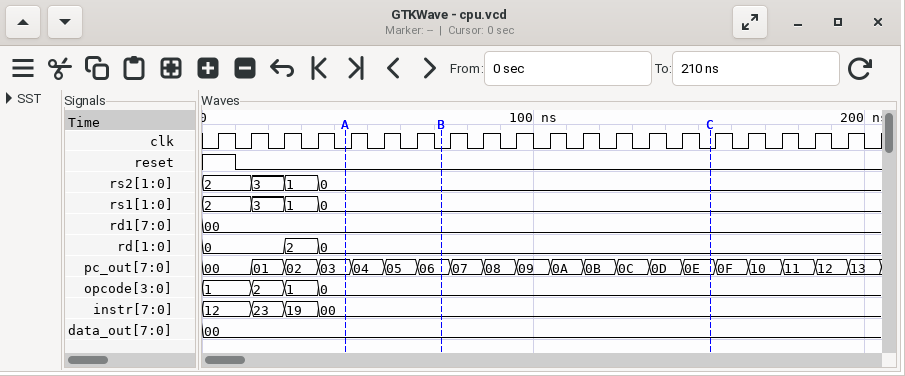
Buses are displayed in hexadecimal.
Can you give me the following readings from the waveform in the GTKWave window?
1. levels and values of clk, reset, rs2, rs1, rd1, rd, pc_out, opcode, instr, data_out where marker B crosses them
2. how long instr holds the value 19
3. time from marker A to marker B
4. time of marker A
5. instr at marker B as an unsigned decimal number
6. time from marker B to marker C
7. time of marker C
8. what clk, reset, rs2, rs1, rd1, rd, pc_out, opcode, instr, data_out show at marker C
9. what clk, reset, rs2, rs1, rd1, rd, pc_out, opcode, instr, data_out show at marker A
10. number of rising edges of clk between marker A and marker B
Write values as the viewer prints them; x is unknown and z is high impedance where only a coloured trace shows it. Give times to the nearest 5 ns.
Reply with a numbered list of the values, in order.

1. clk=0, reset=0, rs2=0, rs1=0, rd1=00, rd=0, pc_out=06, opcode=0, instr=00, data_out=00
2. 10 ns
3. 30 ns
4. 45 ns
5. 0
6. 80 ns
7. 155 ns
8. clk=0, reset=0, rs2=0, rs1=0, rd1=00, rd=0, pc_out=0E, opcode=0, instr=00, data_out=00
9. clk=0, reset=0, rs2=0, rs1=0, rd1=00, rd=0, pc_out=03, opcode=0, instr=00, data_out=00
10. 3
